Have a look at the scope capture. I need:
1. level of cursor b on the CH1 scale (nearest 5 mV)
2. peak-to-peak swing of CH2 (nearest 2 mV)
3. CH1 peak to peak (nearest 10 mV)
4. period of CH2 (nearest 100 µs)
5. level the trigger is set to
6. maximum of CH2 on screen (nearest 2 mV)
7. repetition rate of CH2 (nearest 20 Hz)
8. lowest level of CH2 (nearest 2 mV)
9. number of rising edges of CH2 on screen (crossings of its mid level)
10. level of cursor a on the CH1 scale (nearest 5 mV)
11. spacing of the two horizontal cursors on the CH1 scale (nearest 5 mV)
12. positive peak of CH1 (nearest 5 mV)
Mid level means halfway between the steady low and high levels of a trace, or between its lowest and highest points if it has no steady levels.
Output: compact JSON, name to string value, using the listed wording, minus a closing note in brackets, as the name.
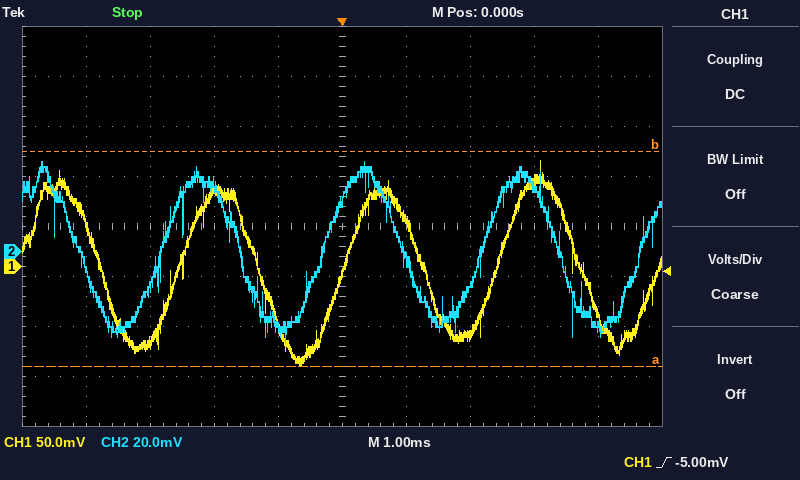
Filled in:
{"level of cursor b on the CH1 scale": "115 mV", "peak-to-peak swing of CH2": "72 mV", "CH1 peak to peak": "200 mV", "period of CH2": "2.5 ms", "level the trigger is set to": "-5.00 mV", "maximum of CH2 on screen": "36 mV", "repetition rate of CH2": "400 Hz", "lowest level of CH2": "-36 mV", "number of rising edges of CH2 on screen": "4", "level of cursor a on the CH1 scale": "-100 mV", "spacing of the two horizontal cursors on the CH1 scale": "215 mV", "positive peak of CH1": "105 mV"}
